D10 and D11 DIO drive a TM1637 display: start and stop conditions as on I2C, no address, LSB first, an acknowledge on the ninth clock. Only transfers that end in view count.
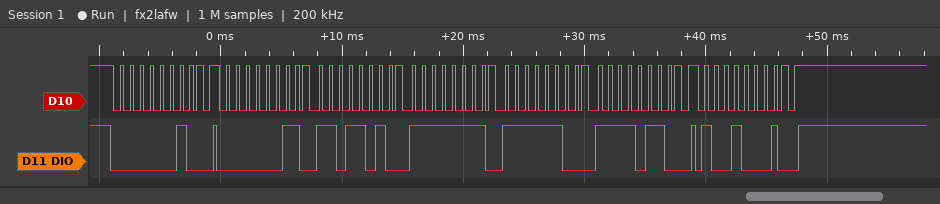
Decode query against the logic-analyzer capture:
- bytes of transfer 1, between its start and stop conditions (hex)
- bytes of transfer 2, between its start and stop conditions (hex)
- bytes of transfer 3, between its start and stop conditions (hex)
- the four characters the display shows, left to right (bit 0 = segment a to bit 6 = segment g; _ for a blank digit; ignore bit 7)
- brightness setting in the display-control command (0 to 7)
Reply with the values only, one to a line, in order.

40
C0 5B FF 3F 6F
89
2809
1
